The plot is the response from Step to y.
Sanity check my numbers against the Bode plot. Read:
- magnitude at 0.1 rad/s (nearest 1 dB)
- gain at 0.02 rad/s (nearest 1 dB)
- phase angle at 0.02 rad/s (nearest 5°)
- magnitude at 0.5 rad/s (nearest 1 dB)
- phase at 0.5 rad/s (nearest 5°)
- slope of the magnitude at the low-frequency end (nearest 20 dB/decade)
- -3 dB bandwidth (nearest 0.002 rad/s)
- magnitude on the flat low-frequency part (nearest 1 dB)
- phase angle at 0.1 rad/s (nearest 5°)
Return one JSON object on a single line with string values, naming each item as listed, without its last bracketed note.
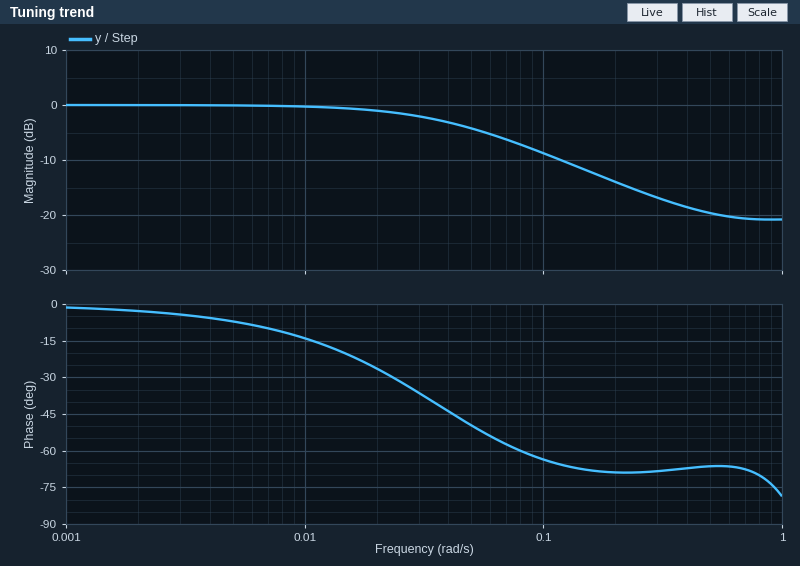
{"magnitude at 0.1 rad/s": "-9 dB", "gain at 0.02 rad/s": "-1 dB", "phase angle at 0.02 rad/s": "-25°", "magnitude at 0.5 rad/s": "-20 dB", "phase at 0.5 rad/s": "-65°", "slope of the magnitude at the low-frequency end": "0 dB/decade", "-3 dB bandwidth": "0.038 rad/s", "magnitude on the flat low-frequency part": "0 dB", "phase angle at 0.1 rad/s": "-65°"}
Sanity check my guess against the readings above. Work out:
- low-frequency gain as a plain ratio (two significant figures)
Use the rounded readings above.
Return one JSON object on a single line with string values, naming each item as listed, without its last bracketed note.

{"low-frequency gain as a plain ratio": "1.0"}
